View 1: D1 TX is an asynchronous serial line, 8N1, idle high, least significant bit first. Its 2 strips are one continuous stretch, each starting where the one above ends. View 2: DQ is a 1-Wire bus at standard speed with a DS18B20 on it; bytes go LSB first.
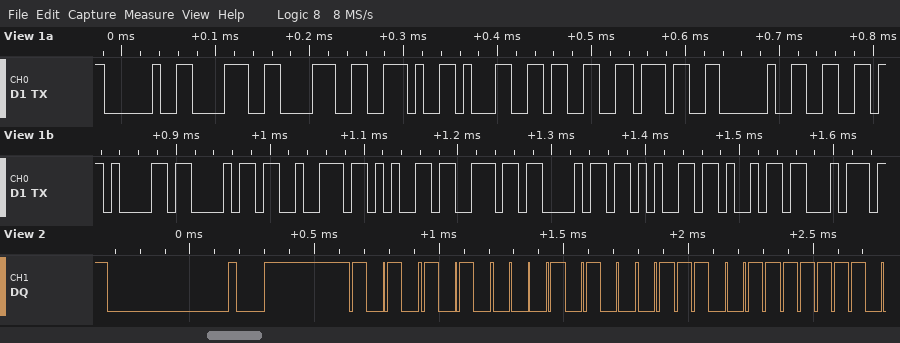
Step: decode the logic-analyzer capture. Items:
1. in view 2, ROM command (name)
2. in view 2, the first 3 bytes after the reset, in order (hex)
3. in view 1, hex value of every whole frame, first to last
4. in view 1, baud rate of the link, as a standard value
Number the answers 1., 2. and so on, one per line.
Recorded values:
1. Match ROM
2. 55 28 CE
3. 0x20 0x38 0x38 0x2E 0x31 0x33 0x37 0x20 0x66 0x61 0x68 0x72 0x65 0x6E 0x68 0x65 0x69 0x74
4. 115200 baud
